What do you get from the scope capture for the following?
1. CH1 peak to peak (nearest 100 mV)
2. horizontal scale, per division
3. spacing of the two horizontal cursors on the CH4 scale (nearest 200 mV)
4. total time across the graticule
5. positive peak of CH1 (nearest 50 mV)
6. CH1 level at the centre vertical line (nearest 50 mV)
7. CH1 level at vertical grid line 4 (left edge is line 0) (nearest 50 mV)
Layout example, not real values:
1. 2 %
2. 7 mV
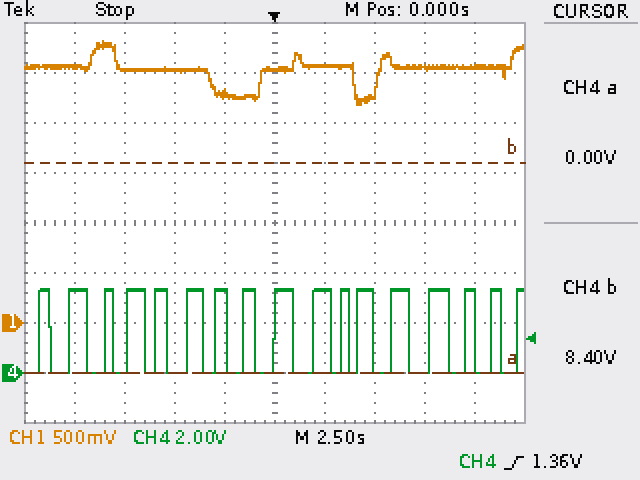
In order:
1. 600 mV
2. 2.5 s
3. 8.4 V
4. 25 s
5. 2.80 V
6. 2.55 V
7. 2.30 V
